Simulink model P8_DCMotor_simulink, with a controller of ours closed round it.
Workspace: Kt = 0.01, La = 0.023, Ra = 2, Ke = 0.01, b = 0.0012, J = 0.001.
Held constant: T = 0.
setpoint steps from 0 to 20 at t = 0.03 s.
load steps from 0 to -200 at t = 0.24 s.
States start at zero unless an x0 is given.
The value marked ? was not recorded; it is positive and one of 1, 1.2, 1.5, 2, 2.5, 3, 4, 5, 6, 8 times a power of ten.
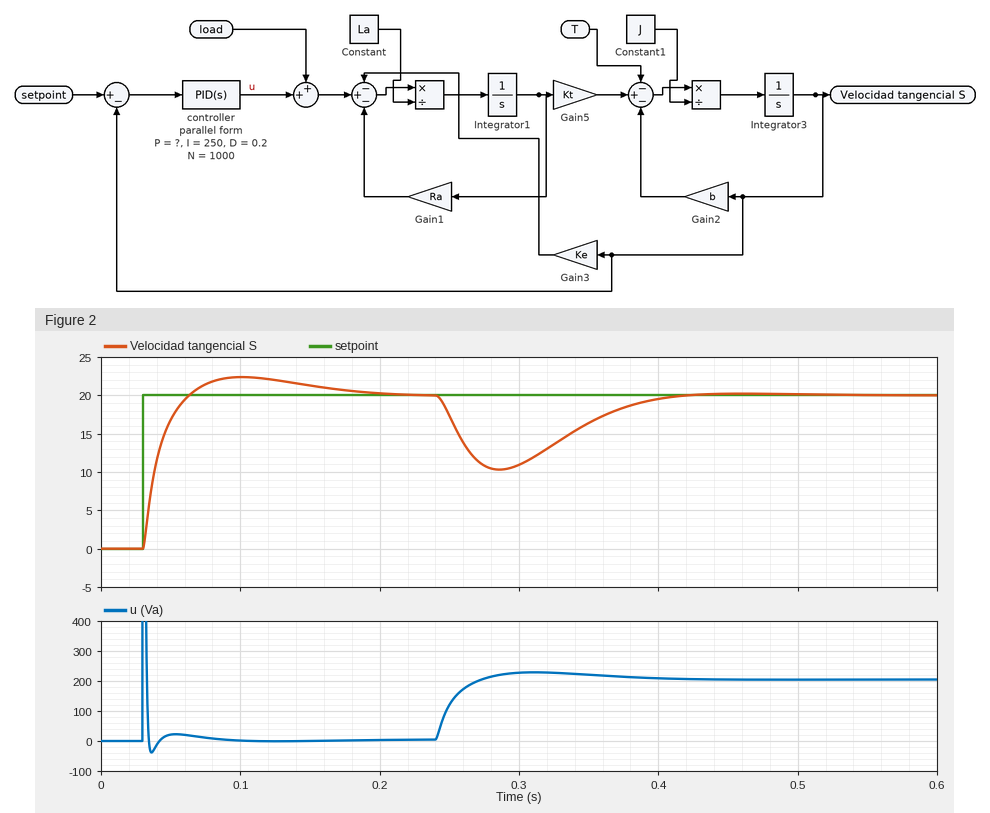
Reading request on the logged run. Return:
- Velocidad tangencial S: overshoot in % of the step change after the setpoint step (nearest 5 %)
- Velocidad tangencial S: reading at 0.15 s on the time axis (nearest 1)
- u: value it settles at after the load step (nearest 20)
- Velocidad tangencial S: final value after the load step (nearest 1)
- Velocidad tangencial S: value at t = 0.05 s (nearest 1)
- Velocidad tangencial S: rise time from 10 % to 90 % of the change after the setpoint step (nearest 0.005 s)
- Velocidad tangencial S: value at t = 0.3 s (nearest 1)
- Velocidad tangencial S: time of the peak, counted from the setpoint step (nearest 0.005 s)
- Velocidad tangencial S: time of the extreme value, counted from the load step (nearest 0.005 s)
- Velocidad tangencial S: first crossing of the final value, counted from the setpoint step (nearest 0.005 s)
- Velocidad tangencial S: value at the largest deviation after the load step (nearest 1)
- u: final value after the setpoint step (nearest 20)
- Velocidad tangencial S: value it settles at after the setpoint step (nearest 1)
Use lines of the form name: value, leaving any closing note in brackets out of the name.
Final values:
Velocidad tangencial S: overshoot in % of the step change after the setpoint step: 10 %
Velocidad tangencial S: reading at 0.15 s on the time axis: 21
u: value it settles at after the load step: 200
Velocidad tangencial S: final value after the load step: 20
Velocidad tangencial S: value at t = 0.05 s: 17
Velocidad tangencial S: rise time from 10 % to 90 % of the change after the setpoint step: 0.020 s
Velocidad tangencial S: value at t = 0.3 s: 11
Velocidad tangencial S: time of the peak, counted from the setpoint step: 0.070 s
Velocidad tangencial S: time of the extreme value, counted from the load step: 0.045 s
Velocidad tangencial S: first crossing of the final value, counted from the setpoint step: 0.035 s
Velocidad tangencial S: value at the largest deviation after the load step: 10
u: final value after the setpoint step: 0
Velocidad tangencial S: value it settles at after the setpoint step: 20
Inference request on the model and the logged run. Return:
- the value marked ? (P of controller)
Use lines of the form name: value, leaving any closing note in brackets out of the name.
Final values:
the value marked ?: 15
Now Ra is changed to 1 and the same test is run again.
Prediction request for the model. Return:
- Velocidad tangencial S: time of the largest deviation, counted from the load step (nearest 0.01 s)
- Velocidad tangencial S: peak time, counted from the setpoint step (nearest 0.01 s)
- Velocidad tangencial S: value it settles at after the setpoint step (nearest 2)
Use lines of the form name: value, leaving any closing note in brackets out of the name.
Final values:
Velocidad tangencial S: time of the largest deviation, counted from the load step: 0.04 s
Velocidad tangencial S: peak time, counted from the setpoint step: 0.04 s
Velocidad tangencial S: value it settles at after the setpoint step: 20
